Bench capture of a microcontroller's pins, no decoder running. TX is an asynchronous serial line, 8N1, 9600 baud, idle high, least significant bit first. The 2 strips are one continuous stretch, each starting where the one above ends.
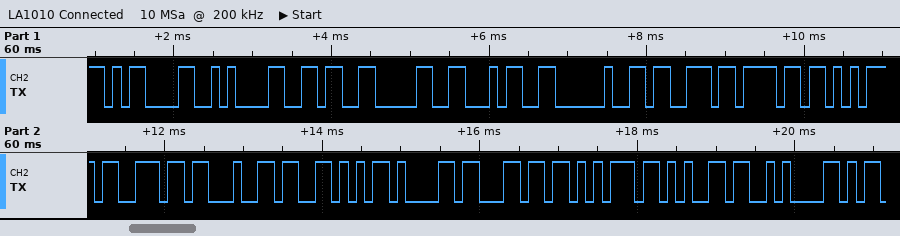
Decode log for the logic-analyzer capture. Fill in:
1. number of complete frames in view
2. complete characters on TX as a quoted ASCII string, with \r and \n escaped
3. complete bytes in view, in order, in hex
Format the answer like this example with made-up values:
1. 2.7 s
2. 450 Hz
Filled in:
1. 17
2. "\r\n604 soundValue\n"
3. 0x0D 0x0A 0x36 0x30 0x34 0x20 0x73 0x6F 0x75 0x6E 0x64 0x56 0x61 0x6C 0x75 0x65 0x0A
